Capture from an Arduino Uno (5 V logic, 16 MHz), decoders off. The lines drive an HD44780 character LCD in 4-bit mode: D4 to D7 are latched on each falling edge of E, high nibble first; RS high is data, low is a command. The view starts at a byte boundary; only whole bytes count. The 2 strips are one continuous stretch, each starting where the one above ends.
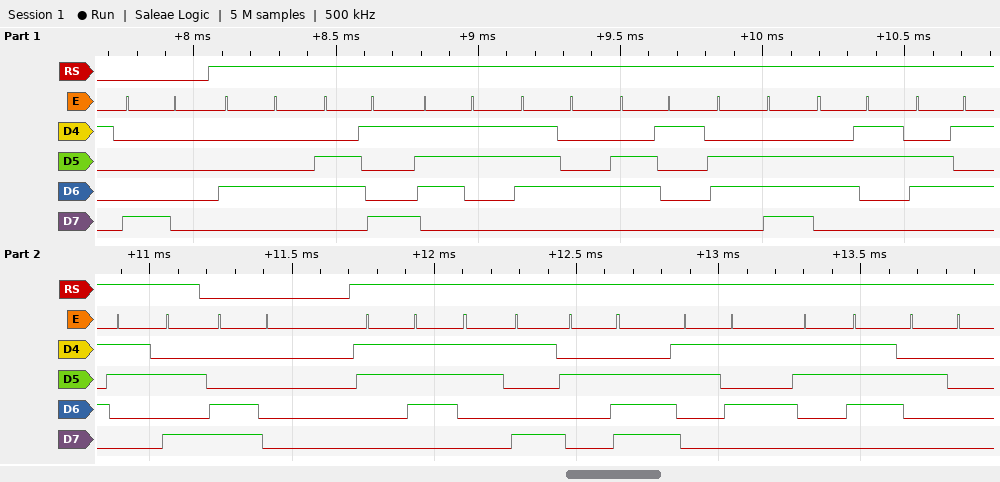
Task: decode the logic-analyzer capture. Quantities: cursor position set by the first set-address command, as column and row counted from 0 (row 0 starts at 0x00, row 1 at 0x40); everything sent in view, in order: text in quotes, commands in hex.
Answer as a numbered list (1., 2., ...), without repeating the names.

1. column 0, row 0
2. 0x80 "Distance:" 0xC0 "79.57 "
